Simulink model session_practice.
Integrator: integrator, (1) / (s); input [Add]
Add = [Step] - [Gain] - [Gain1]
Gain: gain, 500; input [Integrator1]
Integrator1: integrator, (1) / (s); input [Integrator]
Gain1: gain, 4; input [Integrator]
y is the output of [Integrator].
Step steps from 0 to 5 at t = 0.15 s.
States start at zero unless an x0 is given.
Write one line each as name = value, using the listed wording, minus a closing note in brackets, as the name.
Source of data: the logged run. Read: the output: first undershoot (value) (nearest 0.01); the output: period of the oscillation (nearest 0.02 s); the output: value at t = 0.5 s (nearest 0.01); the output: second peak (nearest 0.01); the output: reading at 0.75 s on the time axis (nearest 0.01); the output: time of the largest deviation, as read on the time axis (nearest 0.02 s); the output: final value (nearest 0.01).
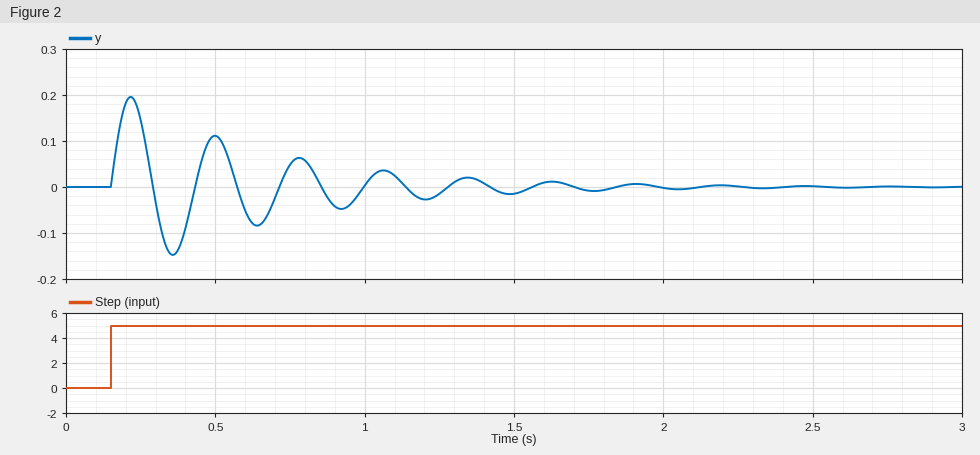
the output: first undershoot (value) = -0.15
the output: period of the oscillation = 0.28 s
the output: value at t = 0.5 s = 0.11
the output: second peak = 0.11
the output: reading at 0.75 s on the time axis = 0.05
the output: time of the largest deviation, as read on the time axis = 0.22 s
the output: final value = 0.00
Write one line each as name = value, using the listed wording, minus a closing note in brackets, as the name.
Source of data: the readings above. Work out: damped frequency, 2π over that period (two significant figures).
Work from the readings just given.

damped frequency, 2π over that period = 22 rad/s
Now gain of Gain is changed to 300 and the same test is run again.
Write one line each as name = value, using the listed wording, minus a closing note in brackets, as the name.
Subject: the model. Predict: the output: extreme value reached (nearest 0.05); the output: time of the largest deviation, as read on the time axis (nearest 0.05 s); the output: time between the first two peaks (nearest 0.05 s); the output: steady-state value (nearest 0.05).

the output: extreme value reached = 0.25
the output: time of the largest deviation, as read on the time axis = 0.25 s
the output: time between the first two peaks = 0.35 s
the output: steady-state value = 0.00
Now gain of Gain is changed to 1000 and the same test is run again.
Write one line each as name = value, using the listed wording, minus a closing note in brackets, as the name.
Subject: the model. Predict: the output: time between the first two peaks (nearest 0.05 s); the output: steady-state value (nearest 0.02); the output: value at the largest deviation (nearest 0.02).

the output: time between the first two peaks = 0.20 s
the output: steady-state value = 0.00
the output: value at the largest deviation = 0.14
